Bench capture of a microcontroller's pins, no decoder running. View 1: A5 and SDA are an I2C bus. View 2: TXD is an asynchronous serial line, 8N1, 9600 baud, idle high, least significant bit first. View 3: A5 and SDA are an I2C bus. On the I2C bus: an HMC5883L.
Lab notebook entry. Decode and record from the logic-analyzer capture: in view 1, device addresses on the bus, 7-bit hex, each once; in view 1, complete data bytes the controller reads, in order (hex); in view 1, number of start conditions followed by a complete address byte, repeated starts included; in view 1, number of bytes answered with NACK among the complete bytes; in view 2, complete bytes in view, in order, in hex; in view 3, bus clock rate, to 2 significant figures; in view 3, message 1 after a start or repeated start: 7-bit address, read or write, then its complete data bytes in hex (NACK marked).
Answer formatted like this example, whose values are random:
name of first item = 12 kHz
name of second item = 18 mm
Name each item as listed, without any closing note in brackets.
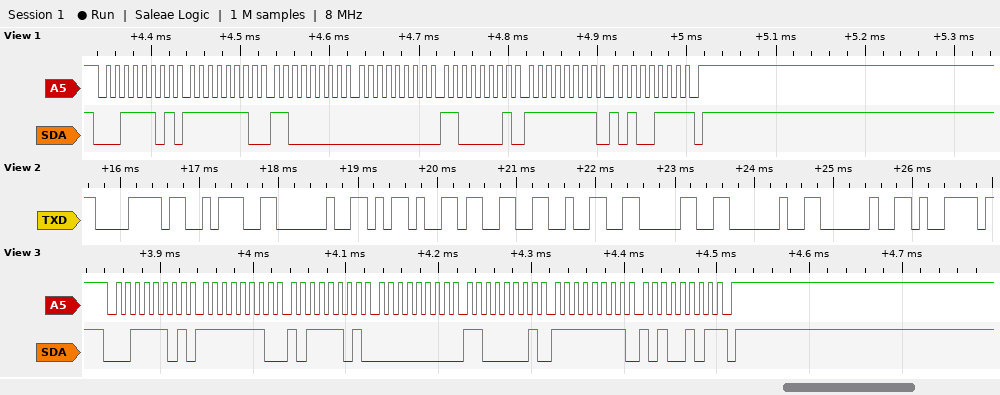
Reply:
in view 1, device addresses on the bus, 7-bit hex, each once = 0x1E
in view 1, complete data bytes the controller reads, in order = FE C0 00 C1 FF A7
in view 1, number of start conditions followed by a complete address byte, repeated starts included = 1
in view 1, number of bytes answered with NACK among the complete bytes = 1
in view 2, complete bytes in view, in order, in hex = 78 3A 20 2D 33 32 30 20 20 79
in view 3, bus clock rate, to 2 significant figures = 100 kHz
in view 3, message 1 after a start or repeated start: 7-bit address, read or write, then its complete data bytes in hex = 0x1E read: FE BD 00 C1 FF A5 NACK
